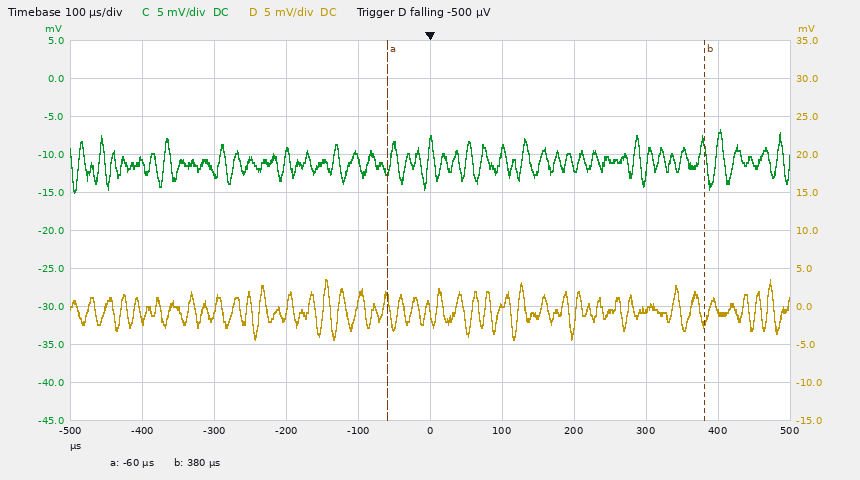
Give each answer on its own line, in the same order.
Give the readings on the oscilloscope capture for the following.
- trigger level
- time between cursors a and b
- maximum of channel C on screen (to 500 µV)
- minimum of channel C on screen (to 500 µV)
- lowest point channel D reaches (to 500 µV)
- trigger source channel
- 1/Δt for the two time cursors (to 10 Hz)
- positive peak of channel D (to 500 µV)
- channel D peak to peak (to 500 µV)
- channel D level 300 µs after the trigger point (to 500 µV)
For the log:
-500 µV
440 µs
-6.5 mV
-15.0 mV
-4.5 mV
channel D
2.27 kHz
3.5 mV
8.0 mV
-500 µV
